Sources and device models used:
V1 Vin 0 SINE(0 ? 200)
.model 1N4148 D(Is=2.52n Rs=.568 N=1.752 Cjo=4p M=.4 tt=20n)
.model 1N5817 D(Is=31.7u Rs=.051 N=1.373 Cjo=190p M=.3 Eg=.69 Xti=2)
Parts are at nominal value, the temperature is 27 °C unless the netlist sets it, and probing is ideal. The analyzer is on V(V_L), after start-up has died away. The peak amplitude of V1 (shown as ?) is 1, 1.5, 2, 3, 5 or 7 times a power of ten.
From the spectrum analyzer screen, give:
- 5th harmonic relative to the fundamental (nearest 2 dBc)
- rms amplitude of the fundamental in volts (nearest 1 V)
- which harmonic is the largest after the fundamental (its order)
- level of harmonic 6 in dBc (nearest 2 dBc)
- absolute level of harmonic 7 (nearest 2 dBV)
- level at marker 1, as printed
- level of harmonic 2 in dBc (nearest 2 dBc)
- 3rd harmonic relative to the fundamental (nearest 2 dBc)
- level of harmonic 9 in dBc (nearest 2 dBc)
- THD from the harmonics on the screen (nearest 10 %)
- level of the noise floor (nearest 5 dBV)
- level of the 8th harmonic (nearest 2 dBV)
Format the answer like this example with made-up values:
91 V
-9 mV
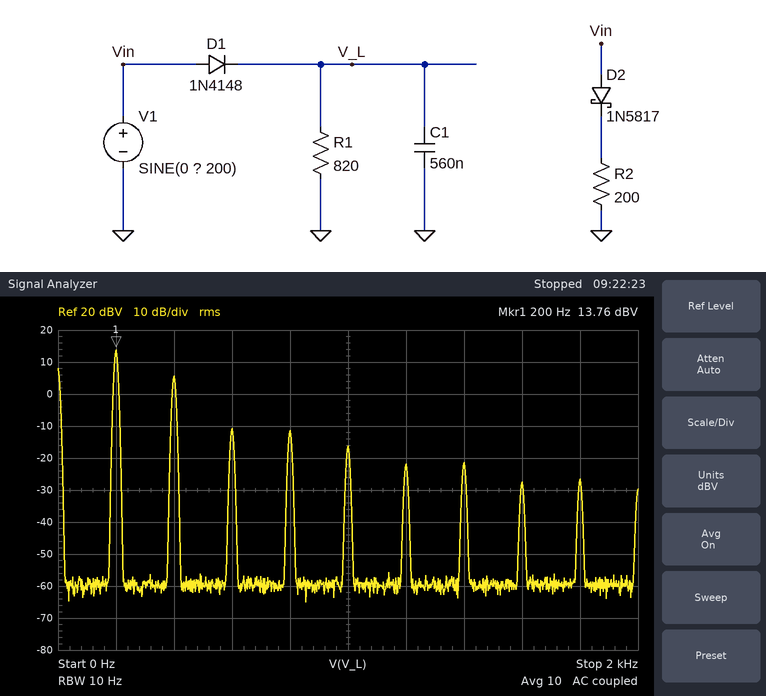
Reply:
-30 dBc
5 V
2
-36 dBc
-22 dBV
13.76 dBV
-8 dBc
-24 dBc
-40 dBc
40 %
-60 dBV
-28 dBV
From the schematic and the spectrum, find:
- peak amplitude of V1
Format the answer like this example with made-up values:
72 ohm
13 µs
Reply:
15 V
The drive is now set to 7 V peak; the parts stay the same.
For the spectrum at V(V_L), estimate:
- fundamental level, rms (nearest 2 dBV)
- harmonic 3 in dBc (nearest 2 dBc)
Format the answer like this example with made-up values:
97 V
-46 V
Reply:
6 dBV
-22 dBc
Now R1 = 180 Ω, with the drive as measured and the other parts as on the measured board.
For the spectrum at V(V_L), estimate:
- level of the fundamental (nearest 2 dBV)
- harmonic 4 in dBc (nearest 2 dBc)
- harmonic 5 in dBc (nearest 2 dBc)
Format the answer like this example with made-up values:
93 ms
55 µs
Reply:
14 dBV
-22 dBc
-38 dBc
